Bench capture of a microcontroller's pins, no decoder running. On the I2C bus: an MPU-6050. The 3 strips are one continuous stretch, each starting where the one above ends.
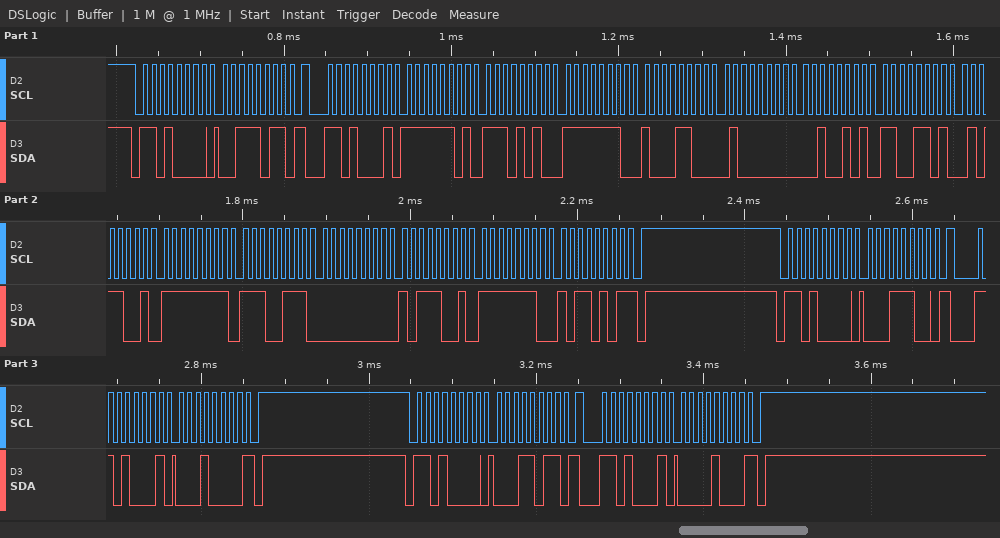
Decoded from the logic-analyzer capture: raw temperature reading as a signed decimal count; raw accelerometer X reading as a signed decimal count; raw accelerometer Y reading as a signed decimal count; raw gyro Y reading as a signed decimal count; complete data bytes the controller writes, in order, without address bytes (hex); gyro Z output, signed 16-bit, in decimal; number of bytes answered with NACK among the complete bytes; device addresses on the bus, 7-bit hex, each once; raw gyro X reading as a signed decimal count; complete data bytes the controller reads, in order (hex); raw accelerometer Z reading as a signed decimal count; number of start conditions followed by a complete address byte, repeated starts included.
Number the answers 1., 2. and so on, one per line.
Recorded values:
1. -12967
2. -534
3. -372
4. 185
5. 3B 1C 1B
6. -331
7. 3
8. 0x68
9. -25
10. FD EA FE 8C 40 25 CD 59 FF E7 00 B9 FE B5 10 08
11. 16421
12. 6
